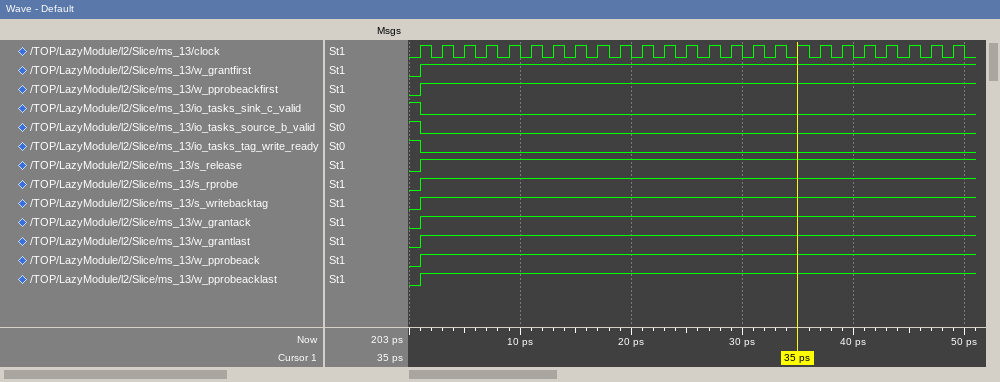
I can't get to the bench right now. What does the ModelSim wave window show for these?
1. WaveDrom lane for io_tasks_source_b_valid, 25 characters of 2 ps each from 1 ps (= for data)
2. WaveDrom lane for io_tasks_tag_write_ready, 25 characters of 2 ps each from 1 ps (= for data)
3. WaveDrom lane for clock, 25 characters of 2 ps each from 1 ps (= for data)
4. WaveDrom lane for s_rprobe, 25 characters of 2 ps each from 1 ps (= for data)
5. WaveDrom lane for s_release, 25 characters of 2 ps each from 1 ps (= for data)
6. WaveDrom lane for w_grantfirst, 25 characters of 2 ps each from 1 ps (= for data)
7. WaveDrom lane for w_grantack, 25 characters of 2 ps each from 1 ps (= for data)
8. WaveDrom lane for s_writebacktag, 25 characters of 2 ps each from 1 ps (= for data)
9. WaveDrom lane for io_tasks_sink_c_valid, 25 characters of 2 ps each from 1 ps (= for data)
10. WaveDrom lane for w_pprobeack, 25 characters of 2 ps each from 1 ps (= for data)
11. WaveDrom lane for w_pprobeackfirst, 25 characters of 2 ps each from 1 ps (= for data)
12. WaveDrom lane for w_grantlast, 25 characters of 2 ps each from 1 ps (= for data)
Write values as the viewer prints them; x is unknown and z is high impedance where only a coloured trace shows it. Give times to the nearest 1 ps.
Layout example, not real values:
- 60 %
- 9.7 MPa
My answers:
- {name: 'io_tasks_source_b_valid', wave: '0........................'}
- {name: 'io_tasks_tag_write_ready', wave: '0........................'}
- {name: 'clock', wave: 'p........................'}
- {name: 's_rprobe', wave: '1........................'}
- {name: 's_release', wave: '1........................'}
- {name: 'w_grantfirst', wave: '1........................'}
- {name: 'w_grantack', wave: '1........................'}
- {name: 's_writebacktag', wave: '1........................'}
- {name: 'io_tasks_sink_c_valid', wave: '0........................'}
- {name: 'w_pprobeack', wave: '1........................'}
- {name: 'w_pprobeackfirst', wave: '1........................'}
- {name: 'w_grantlast', wave: '1........................'}
